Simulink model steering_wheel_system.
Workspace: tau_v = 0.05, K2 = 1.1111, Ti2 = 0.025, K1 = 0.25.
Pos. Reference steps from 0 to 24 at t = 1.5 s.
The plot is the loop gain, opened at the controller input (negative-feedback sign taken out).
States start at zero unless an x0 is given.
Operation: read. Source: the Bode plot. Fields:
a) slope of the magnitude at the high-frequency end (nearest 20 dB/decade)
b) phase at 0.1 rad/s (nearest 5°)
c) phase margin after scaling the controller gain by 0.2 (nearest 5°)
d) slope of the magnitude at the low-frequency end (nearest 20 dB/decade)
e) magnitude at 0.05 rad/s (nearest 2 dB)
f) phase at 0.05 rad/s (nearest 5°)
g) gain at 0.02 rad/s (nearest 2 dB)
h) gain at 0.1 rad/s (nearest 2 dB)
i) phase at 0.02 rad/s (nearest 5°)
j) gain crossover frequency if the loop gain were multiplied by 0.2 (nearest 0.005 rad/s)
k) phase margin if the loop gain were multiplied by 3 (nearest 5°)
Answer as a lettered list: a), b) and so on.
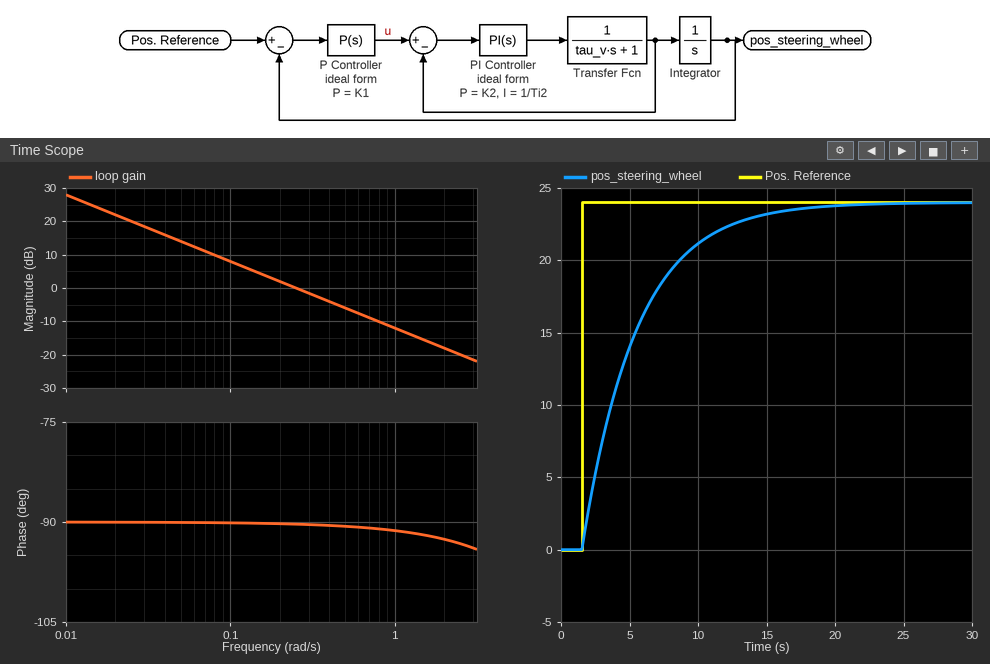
a) -20 dB/decade
b) -90°
c) 90°
d) -20 dB/decade
e) 14 dB
f) -90°
g) 22 dB
h) 8 dB
i) -90°
j) 0.050 rad/s
k) 90°
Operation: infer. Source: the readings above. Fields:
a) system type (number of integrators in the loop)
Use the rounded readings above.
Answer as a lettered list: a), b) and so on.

a) 1
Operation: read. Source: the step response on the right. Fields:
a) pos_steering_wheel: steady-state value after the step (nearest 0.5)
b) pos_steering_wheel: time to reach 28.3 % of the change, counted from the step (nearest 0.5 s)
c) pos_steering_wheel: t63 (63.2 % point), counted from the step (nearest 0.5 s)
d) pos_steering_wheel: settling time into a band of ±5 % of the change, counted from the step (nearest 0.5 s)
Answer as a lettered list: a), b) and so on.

a) 24.0
b) 1.5 s
c) 4.0 s
d) 12.0 s
